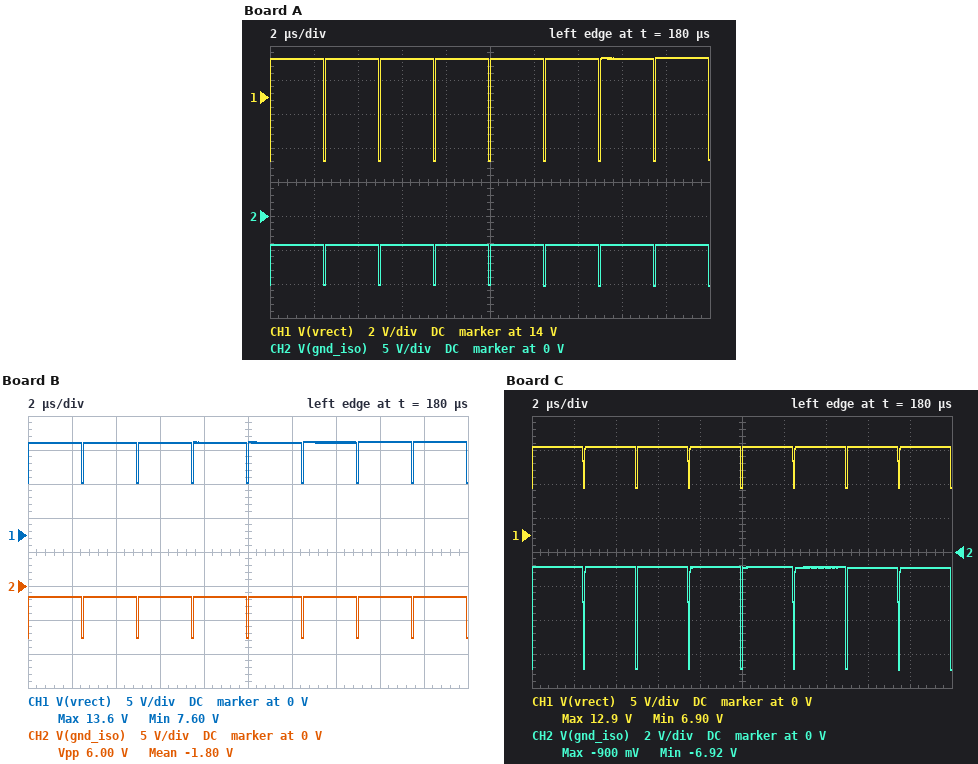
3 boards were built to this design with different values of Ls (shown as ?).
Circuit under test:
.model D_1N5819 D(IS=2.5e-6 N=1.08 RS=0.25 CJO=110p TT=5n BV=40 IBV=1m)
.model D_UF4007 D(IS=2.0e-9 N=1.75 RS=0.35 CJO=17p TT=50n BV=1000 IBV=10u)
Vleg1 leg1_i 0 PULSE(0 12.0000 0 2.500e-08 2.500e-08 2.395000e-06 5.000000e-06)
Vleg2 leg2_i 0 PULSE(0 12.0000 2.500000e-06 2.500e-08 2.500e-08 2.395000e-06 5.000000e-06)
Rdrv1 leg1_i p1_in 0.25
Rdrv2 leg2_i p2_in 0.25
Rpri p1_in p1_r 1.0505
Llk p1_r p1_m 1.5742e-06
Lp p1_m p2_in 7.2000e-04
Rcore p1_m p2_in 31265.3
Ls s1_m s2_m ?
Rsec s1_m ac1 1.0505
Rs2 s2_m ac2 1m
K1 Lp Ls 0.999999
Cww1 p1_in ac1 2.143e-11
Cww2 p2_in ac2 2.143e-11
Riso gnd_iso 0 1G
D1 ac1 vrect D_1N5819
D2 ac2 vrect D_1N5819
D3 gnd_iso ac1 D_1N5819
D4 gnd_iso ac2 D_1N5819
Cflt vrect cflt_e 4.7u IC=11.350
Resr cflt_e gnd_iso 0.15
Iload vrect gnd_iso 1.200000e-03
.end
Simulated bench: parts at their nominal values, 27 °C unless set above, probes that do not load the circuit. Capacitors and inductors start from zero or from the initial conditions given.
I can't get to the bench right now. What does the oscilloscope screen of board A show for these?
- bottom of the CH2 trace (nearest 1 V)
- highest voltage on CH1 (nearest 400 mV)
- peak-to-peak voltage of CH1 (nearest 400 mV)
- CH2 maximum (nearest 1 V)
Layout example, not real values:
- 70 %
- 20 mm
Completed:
- -10 V
- 16.4 V
- 6.0 V
- -4 V
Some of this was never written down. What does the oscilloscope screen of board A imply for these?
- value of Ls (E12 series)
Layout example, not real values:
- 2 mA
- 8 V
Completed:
- 2.2 mH
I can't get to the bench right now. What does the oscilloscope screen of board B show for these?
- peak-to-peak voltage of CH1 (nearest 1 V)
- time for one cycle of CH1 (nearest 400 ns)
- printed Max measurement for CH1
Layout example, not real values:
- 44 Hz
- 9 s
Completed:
- 6 V
- 2.4 µs
- 13.6 V
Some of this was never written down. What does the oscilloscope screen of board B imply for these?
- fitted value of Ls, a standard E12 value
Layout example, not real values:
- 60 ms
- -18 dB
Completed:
- 1.2 mH
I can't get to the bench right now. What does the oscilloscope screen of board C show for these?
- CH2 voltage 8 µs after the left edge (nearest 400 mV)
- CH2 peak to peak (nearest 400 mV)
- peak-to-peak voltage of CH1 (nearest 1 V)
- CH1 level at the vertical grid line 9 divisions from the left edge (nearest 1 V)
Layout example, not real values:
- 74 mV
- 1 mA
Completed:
- -800 mV
- 6.0 V
- 6 V
- 13 V
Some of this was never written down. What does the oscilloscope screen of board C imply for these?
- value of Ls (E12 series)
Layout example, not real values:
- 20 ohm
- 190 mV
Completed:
- 1 mH
